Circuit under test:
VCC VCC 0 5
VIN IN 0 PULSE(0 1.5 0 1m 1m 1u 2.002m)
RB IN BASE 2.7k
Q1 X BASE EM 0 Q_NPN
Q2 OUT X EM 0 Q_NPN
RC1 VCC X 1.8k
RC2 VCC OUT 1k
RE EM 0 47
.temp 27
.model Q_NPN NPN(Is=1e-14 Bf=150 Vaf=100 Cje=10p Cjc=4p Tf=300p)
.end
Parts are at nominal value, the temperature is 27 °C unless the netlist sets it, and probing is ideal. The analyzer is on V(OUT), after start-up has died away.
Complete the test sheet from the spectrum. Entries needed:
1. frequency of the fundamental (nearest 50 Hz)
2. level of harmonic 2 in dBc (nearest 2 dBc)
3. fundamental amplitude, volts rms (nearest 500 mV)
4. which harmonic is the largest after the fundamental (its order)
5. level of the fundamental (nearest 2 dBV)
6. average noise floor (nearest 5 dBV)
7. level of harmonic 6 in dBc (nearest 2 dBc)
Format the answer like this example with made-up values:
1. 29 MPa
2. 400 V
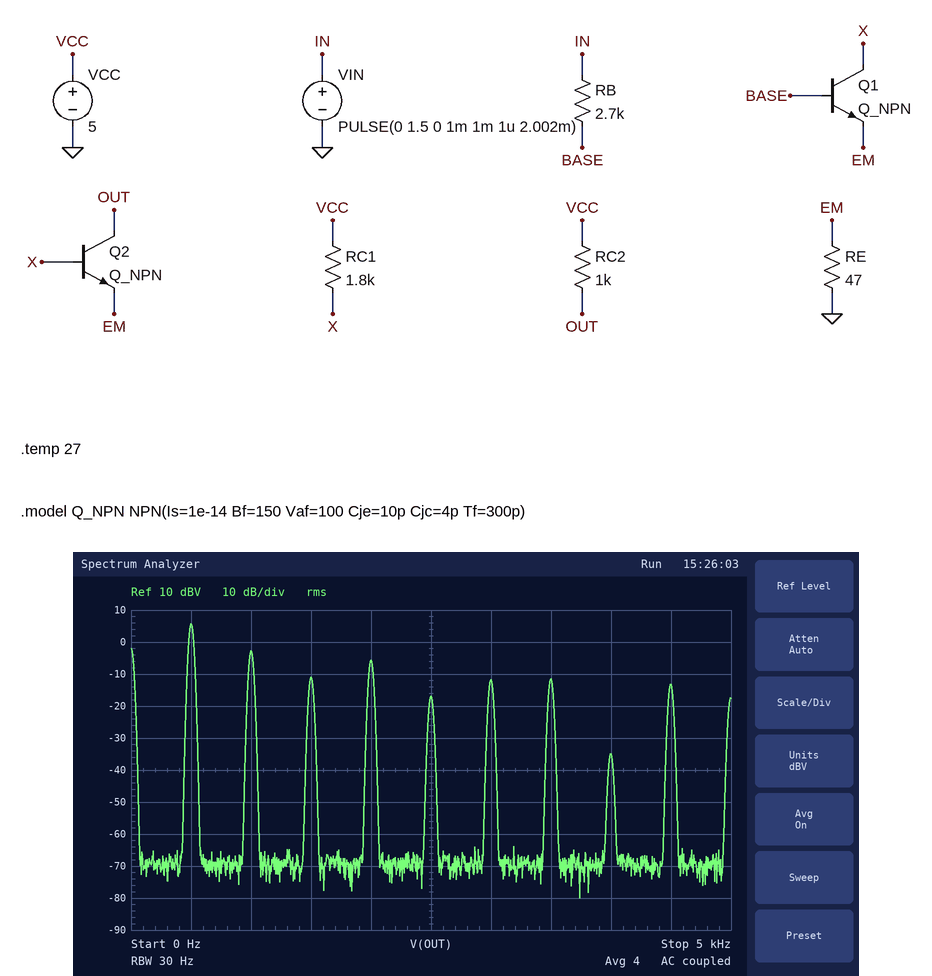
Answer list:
1. 500 Hz
2. -8 dBc
3. 2.0 V
4. 2
5. 6 dBV
6. -70 dBV
7. -18 dBc
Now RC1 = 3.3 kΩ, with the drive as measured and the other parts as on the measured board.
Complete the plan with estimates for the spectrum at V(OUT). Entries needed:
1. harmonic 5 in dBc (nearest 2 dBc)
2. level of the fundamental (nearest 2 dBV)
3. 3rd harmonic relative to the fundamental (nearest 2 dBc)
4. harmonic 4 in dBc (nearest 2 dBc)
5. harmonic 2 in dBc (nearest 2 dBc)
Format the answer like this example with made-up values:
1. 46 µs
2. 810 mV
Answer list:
1. -20 dBc
2. 6 dBV
3. -12 dBc
4. -14 dBc
5. -14 dBc
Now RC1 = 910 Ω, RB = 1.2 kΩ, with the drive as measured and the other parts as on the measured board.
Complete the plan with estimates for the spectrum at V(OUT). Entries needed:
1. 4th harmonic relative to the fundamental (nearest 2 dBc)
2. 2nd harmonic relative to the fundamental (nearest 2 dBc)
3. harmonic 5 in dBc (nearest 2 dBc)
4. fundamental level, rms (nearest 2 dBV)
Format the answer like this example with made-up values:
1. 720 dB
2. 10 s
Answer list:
1. -14 dBc
2. -4 dBc
3. -12 dBc
4. 4 dBV
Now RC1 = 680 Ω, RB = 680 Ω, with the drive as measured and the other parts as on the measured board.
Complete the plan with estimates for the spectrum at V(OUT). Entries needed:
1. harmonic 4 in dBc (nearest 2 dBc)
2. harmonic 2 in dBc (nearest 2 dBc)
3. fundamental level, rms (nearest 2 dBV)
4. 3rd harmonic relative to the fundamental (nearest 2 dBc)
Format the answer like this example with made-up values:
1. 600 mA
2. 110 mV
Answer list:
1. -26 dBc
2. -4 dBc
3. 4 dBV
4. -10 dBc
